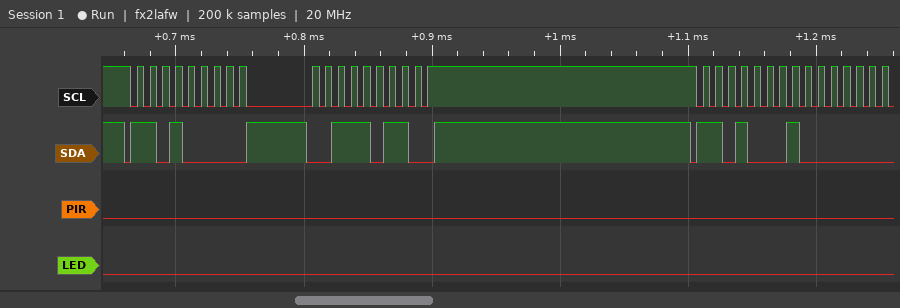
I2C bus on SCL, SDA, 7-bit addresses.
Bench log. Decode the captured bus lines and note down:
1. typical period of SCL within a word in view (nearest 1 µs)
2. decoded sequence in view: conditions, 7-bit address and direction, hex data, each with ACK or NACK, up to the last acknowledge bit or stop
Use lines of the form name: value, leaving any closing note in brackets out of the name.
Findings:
typical period of SCL within a word in view: 10 µs
decoded sequence in view: conditions, 7-bit address and direction, hex data, each with ACK or NACK, up to the last acknowledge bit or stop: start, address 68 write ACK, 3B ACK, stop, start, address 68 read ACK
